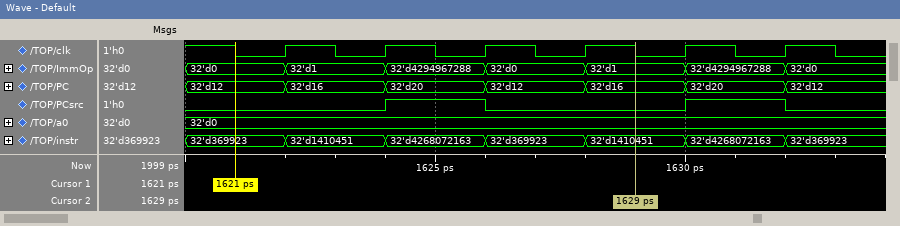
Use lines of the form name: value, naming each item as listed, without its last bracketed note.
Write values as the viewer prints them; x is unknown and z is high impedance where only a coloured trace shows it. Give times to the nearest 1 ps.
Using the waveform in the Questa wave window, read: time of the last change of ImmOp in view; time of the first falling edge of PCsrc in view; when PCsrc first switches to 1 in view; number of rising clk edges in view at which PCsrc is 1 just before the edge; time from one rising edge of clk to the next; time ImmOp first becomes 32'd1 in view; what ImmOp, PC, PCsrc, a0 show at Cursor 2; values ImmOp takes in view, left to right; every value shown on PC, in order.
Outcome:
time of the last change of ImmOp in view: 1632 ps
time of the first falling edge of PCsrc in view: 1626 ps
when PCsrc first switches to 1 in view: 1624 ps
number of rising clk edges in view at which PCsrc is 1 just before the edge: 2
time from one rising edge of clk to the next: 2 ps
time ImmOp first becomes 32'd1 in view: 1622 ps
what ImmOp, PC, PCsrc, a0 show at Cursor 2: ImmOp=32'd1, PC=32'd16, PCsrc=0, a0=32'd0
values ImmOp takes in view, left to right: 32'd0, 32'd1, 32'd4294967288, 32'd0, 32'd1, 32'd4294967288, 32'd0
every value shown on PC, in order: 32'd12, 32'd16, 32'd20, 32'd12, 32'd16, 32'd20, 32'd12
